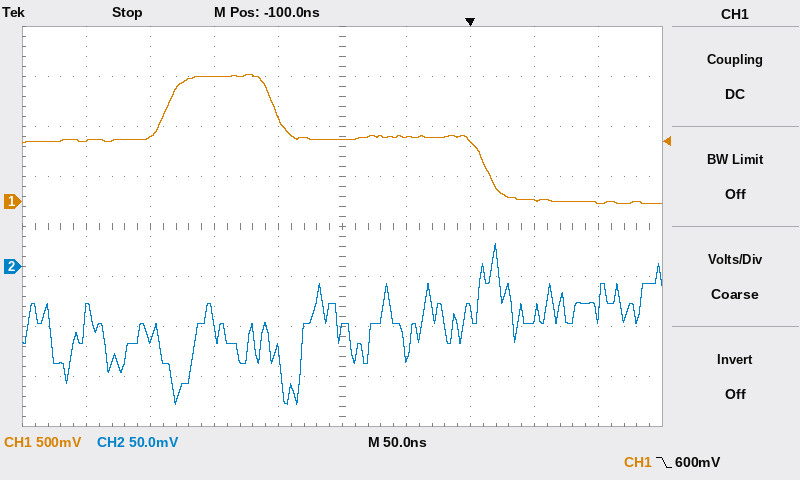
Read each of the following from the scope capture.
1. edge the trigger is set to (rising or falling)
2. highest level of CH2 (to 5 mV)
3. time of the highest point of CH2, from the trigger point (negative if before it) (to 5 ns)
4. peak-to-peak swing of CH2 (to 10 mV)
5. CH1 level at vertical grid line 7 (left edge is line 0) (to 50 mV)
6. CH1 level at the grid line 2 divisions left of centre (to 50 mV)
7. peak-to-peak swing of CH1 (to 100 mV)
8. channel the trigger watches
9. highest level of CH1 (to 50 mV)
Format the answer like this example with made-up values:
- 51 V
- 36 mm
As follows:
- falling
- 25 mV
- +20 ns
- 160 mV
- 600 mV
- 1.25 V
- 1.30 V
- CH1
- 1.25 V
